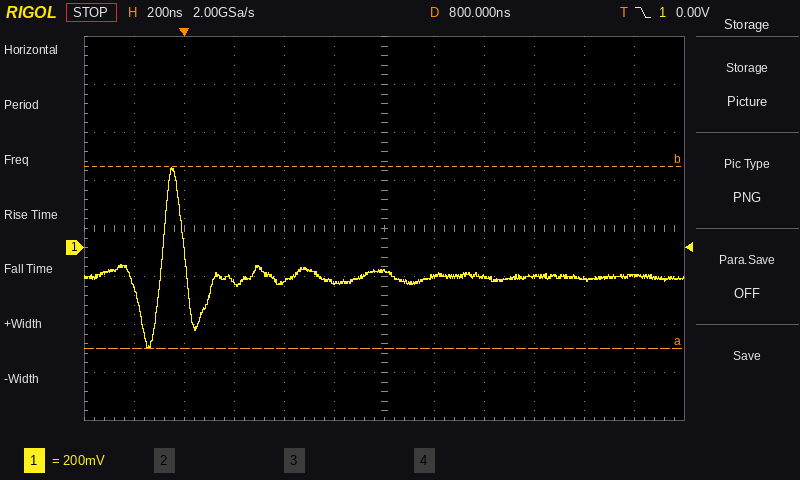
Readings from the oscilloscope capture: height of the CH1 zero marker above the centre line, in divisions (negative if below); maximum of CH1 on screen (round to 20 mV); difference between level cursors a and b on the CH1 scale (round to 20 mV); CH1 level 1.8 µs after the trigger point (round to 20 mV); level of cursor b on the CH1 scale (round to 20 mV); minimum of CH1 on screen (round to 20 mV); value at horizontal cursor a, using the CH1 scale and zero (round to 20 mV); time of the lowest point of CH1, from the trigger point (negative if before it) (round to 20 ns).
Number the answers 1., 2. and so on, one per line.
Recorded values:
1. -0.4 div
2. 340 mV
3. 760 mV
4. -120 mV
5. 340 mV
6. -420 mV
7. -420 mV
8. -140 ns
